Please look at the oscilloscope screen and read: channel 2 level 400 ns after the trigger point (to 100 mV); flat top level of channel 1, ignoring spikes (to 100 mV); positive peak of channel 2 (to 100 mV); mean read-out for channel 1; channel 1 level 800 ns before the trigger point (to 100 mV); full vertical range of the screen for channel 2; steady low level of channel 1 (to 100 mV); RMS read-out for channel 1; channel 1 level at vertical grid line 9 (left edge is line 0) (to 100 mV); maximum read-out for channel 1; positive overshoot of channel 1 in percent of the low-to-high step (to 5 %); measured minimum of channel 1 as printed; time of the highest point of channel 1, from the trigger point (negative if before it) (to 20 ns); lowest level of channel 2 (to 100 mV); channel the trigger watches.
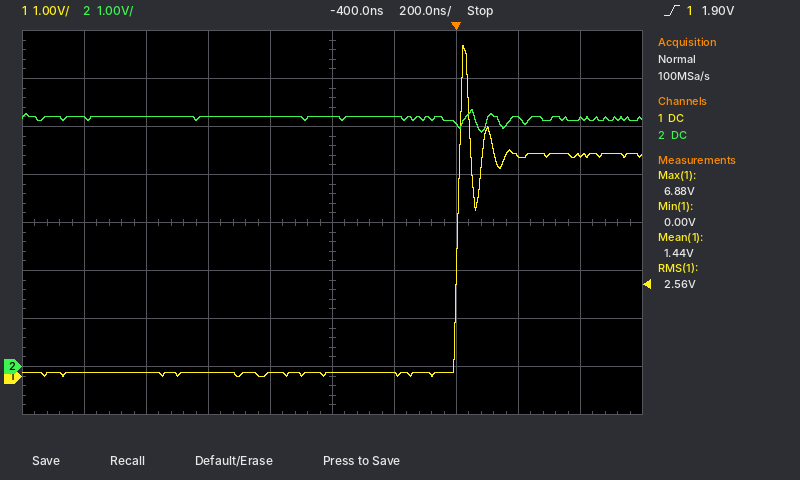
5.2 V
4.6 V
5.4 V
1.44 V
100 mV
8 V
100 mV
2.56 V
4.6 V
6.88 V
50 %
0.00 V
+20 ns
4.9 V
channel 1
